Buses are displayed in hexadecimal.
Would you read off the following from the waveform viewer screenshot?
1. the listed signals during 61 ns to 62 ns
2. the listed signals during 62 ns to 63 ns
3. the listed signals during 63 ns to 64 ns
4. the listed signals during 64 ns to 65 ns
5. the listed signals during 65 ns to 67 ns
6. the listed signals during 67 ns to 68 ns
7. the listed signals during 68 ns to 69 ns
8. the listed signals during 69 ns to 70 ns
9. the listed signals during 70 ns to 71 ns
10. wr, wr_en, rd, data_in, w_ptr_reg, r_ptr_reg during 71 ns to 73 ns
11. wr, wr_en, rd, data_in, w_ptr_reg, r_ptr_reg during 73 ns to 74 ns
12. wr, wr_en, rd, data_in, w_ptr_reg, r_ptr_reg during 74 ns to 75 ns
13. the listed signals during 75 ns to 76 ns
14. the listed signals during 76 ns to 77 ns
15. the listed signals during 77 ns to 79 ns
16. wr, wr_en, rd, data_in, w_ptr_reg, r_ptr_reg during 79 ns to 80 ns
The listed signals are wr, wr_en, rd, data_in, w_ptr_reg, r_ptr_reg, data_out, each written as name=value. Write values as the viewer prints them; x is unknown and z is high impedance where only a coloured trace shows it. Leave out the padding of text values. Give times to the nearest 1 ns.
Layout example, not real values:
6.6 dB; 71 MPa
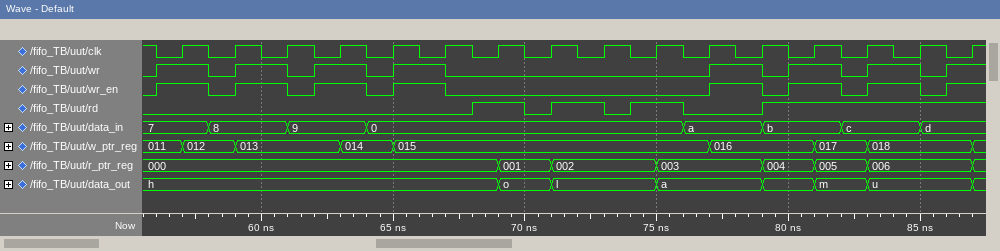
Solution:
wr=0, wr_en=0, rd=0, data_in=9, w_ptr_reg=013, r_ptr_reg=000, data_out=h; wr=1, wr_en=1, rd=0, data_in=9, w_ptr_reg=013, r_ptr_reg=000, data_out=h; wr=1, wr_en=1, rd=0, data_in=9, w_ptr_reg=014, r_ptr_reg=000, data_out=h; wr=0, wr_en=0, rd=0, data_in=0, w_ptr_reg=014, r_ptr_reg=000, data_out=h; wr=1, wr_en=1, rd=0, data_in=0, w_ptr_reg=015, r_ptr_reg=000, data_out=h; wr=0, wr_en=0, rd=0, data_in=0, w_ptr_reg=015, r_ptr_reg=000, data_out=h; wr=0, wr_en=0, rd=1, data_in=0, w_ptr_reg=015, r_ptr_reg=000, data_out=h; wr=0, wr_en=0, rd=1, data_in=0, w_ptr_reg=015, r_ptr_reg=001, data_out=o; wr=0, wr_en=0, rd=0, data_in=0, w_ptr_reg=015, r_ptr_reg=001, data_out=o; wr=0, wr_en=0, rd=1, data_in=0, w_ptr_reg=015, r_ptr_reg=002; wr=0, wr_en=0, rd=0, data_in=0, w_ptr_reg=015, r_ptr_reg=002; wr=0, wr_en=0, rd=1, data_in=0, w_ptr_reg=015, r_ptr_reg=002; wr=0, wr_en=0, rd=1, data_in=0, w_ptr_reg=015, r_ptr_reg=003, data_out=a; wr=0, wr_en=0, rd=0, data_in=a, w_ptr_reg=015, r_ptr_reg=003, data_out=a; wr=1, wr_en=1, rd=0, data_in=a, w_ptr_reg=016, r_ptr_reg=003, data_out=a; wr=0, wr_en=0, rd=1, data_in=b, w_ptr_reg=016, r_ptr_reg=004
